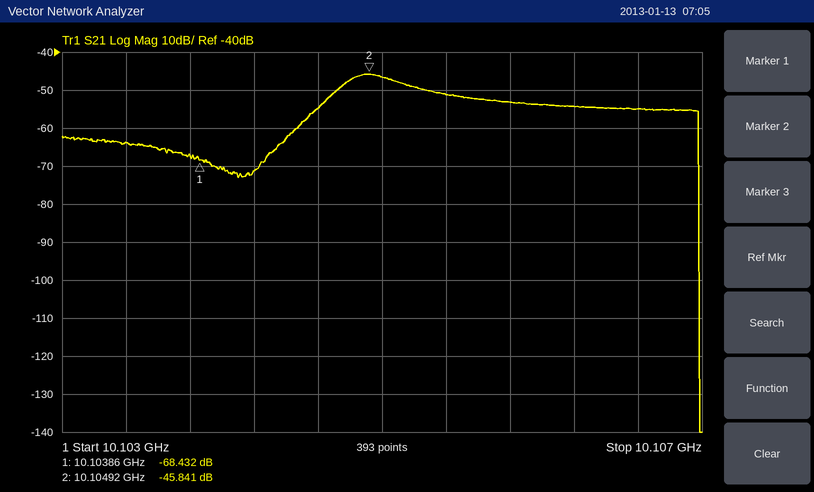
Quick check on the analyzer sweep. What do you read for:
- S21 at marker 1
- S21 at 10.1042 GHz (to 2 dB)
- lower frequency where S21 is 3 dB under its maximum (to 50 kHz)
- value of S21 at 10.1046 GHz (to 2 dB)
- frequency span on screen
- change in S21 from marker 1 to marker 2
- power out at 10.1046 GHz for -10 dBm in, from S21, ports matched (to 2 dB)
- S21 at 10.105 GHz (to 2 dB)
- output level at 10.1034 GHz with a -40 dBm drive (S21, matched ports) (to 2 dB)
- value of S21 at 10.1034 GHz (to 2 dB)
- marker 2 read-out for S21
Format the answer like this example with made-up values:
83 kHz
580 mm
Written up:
-68.432 dB
-72 dB
10.10475 GHz
-54 dB
4 MHz
22.591 dB
-64 dBm
-46 dB
-104 dBm
-64 dB
-45.841 dB
